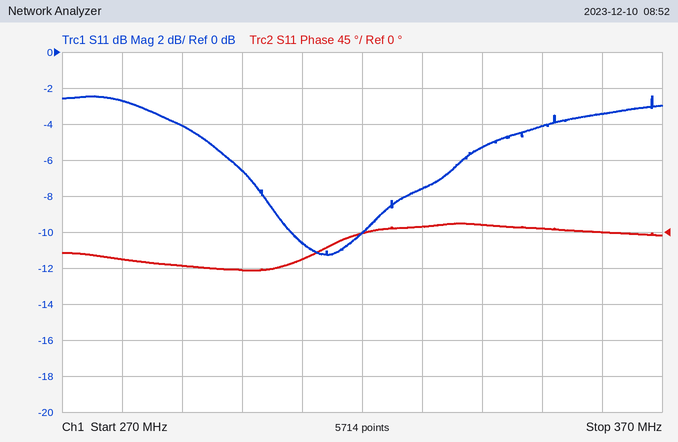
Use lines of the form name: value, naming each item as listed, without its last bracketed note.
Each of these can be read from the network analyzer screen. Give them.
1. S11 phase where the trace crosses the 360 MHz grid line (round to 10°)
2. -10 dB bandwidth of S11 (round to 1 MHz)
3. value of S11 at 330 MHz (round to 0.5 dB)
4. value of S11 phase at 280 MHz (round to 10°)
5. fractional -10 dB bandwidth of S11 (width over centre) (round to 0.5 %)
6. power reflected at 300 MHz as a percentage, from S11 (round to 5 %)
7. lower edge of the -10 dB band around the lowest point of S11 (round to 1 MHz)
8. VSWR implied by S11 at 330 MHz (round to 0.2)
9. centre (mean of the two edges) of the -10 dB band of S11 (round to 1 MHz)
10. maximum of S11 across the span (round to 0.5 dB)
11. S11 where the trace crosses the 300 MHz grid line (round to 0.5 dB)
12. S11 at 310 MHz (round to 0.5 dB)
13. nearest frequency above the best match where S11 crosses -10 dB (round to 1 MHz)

S11 phase where the trace crosses the 360 MHz grid line: 0°
-10 dB bandwidth of S11: 12 MHz
value of S11 at 330 MHz: -7.5 dB
value of S11 phase at 280 MHz: -30°
fractional -10 dB bandwidth of S11 (width over centre): 4.0 %
power reflected at 300 MHz as a percentage, from S11: 20 %
lower edge of the -10 dB band around the lowest point of S11: 308 MHz
VSWR implied by S11 at 330 MHz: 2.4
centre (mean of the two edges) of the -10 dB band of S11: 314 MHz
maximum of S11 across the span: -2.5 dB
S11 where the trace crosses the 300 MHz grid line: -6.5 dB
S11 at 310 MHz: -10.5 dB
nearest frequency above the best match where S11 crosses -10 dB: 320 MHz
